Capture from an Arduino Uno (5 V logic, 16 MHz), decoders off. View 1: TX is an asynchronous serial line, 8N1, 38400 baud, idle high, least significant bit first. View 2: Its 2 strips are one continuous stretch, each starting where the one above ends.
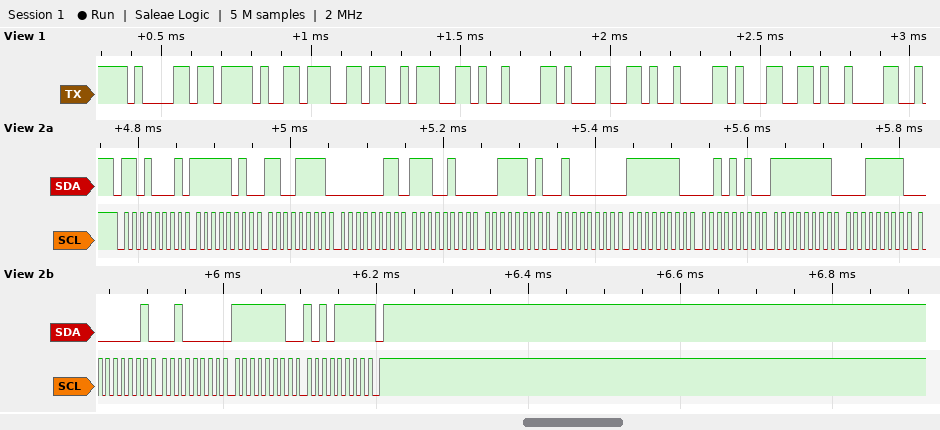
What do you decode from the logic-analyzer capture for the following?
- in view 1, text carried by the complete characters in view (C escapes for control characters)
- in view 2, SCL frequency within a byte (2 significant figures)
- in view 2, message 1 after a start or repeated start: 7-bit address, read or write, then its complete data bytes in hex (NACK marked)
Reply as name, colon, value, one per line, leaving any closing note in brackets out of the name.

in view 1, text carried by the complete characters in view: "a/g:\t1\t1\t"
in view 2, SCL frequency within a byte: 100 kHz
in view 2, message 1 after a start or repeated start: 7-bit address, read or write, then its complete data bytes in hex: 0x68 read: FA CF 03 E4 3D 40 FE 2A FF 1F 01 20 FE AF NACK
